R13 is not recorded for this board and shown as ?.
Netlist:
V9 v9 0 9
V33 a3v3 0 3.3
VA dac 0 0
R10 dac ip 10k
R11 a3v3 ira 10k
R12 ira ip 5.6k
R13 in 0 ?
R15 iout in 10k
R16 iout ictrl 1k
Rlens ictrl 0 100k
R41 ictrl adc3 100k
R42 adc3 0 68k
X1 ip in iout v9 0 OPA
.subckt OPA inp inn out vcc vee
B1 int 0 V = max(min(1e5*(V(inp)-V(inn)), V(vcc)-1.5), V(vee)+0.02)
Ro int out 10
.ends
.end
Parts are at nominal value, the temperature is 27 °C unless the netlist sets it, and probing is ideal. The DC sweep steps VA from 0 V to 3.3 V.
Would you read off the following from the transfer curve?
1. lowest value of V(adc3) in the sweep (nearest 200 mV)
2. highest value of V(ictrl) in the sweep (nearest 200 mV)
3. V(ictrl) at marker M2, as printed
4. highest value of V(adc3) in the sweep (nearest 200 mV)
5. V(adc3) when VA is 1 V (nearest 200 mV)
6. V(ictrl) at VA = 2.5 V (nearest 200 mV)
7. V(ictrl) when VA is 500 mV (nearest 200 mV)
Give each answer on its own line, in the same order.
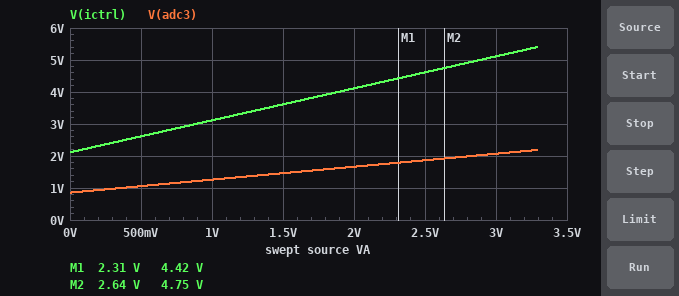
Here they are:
800 mV
5.4 V
4.75 V
2.2 V
1.2 V
4.6 V
2.6 V
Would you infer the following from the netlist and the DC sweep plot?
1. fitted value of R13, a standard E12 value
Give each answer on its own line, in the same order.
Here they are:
15 kΩ
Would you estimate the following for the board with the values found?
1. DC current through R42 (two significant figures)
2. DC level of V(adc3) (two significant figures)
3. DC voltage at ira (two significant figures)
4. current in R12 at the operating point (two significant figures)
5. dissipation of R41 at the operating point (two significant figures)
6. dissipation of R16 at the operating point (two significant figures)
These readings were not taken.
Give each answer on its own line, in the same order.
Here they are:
13 µA
860 mV
2.0 V
130 µA
16 µW
1.1 µW
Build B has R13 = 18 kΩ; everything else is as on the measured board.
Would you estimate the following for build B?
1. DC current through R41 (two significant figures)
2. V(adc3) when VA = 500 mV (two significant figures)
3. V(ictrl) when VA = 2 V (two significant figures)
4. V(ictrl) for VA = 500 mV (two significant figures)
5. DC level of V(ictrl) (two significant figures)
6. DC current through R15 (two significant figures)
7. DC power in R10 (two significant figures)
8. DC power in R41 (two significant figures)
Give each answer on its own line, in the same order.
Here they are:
12 µA
990 mV
3.8 V
2.4 V
2.0 V
72 µA
170 µW
14 µW
